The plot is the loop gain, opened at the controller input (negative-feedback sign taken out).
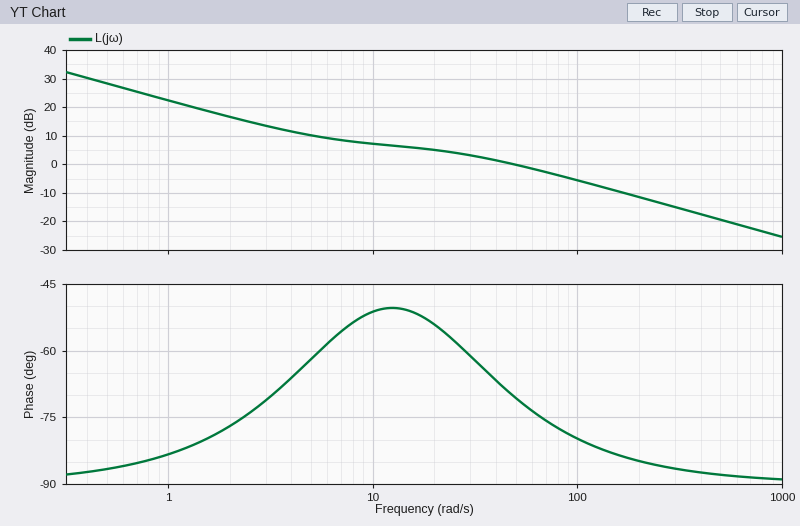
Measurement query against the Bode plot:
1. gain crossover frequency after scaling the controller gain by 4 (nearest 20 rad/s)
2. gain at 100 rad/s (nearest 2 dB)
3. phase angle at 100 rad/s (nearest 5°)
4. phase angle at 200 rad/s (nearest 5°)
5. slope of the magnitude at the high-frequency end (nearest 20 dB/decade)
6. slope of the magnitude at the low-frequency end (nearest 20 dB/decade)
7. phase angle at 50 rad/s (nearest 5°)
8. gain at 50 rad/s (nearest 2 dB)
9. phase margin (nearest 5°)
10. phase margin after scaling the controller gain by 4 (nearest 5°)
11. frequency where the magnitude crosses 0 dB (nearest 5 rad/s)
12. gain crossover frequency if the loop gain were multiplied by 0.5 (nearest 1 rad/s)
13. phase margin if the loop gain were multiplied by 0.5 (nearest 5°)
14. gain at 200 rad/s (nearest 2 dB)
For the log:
220 rad/s
-6 dB
-80°
-85°
-20 dB/decade
-20 dB/decade
-70°
0 dB
110°
95°
50 rad/s
15 rad/s
130°
-12 dB
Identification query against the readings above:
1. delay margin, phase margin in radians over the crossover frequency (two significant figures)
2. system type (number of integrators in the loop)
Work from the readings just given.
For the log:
0.038 s
1
